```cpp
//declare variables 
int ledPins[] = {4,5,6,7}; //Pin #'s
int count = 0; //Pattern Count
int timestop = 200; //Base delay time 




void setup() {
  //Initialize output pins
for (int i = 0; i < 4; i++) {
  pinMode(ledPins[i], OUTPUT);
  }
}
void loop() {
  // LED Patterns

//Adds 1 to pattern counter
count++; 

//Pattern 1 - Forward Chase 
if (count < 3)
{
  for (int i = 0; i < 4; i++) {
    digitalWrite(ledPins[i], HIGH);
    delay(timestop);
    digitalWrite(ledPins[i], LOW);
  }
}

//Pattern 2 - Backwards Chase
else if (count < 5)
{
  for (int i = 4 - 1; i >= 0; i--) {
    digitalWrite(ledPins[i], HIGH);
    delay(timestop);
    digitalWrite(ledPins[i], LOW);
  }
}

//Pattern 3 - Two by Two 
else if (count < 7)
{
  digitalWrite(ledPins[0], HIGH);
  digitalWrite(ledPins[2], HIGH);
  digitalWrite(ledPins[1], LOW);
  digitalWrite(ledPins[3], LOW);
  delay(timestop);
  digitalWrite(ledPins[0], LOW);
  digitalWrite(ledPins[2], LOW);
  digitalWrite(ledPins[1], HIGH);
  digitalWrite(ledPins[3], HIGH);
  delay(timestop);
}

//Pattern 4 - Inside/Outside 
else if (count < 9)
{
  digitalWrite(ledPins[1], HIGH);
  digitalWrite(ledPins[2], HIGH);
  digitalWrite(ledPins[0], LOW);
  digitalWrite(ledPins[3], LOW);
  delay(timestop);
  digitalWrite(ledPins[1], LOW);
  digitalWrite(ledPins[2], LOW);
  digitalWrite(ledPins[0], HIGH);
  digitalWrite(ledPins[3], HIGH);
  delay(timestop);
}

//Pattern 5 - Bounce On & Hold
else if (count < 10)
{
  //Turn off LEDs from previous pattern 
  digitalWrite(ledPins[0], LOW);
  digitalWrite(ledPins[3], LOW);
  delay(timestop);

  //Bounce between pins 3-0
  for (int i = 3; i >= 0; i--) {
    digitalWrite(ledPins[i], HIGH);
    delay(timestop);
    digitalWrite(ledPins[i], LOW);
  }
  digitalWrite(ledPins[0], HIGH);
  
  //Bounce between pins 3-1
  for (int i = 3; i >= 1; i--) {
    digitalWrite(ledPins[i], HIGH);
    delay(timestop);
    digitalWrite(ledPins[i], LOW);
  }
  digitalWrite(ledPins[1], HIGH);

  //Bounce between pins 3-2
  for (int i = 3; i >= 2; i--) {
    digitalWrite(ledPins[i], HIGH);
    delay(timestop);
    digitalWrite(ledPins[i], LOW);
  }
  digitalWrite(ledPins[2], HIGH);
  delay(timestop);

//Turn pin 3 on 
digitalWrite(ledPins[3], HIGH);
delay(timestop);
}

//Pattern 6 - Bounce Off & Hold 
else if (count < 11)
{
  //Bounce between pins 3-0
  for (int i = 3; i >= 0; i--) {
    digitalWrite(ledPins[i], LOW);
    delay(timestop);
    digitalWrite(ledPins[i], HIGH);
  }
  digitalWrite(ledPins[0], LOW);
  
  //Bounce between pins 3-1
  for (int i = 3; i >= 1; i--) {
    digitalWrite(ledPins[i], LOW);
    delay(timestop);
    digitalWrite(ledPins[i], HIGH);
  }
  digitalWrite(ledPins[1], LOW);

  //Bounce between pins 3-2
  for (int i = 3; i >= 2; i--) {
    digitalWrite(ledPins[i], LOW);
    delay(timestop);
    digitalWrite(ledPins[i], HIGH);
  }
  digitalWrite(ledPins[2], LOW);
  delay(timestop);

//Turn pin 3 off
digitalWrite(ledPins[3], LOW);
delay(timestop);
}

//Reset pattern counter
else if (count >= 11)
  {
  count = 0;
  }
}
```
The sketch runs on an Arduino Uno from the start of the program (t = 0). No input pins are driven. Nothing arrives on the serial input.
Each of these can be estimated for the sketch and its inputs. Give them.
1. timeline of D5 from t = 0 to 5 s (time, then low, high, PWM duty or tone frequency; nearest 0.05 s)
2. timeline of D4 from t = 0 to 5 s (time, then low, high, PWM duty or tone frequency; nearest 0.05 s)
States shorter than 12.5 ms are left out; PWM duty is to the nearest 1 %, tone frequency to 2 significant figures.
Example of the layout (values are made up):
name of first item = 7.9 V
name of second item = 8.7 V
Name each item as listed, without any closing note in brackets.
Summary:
timeline of D5 from t = 0 to 5 s = 0 s low; 0.2 s high; 0.4 s low; 1 s high; 1.2 s low; 2 s high; 2.2 s low; 2.8 s high; 3 s low; 3.4 s high; 3.6 s low; 3.8 s high; 4.2 s low; 4.4 s high; 4.6 s low
timeline of D4 from t = 0 to 5 s = 0 s high; 0.2 s low; 0.8 s high; 1 s low; 2.2 s high; 2.4 s low; 3 s high; 3.4 s low; 3.6 s high; 3.8 s low; 4.2 s high; 4.4 s low; 4.6 s high; 4.8 s low
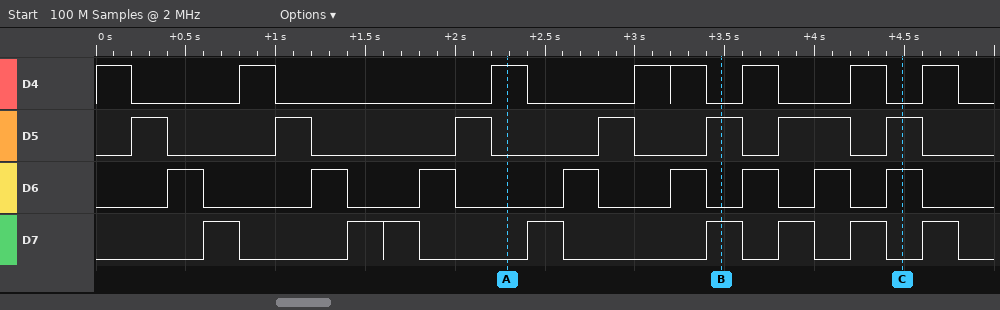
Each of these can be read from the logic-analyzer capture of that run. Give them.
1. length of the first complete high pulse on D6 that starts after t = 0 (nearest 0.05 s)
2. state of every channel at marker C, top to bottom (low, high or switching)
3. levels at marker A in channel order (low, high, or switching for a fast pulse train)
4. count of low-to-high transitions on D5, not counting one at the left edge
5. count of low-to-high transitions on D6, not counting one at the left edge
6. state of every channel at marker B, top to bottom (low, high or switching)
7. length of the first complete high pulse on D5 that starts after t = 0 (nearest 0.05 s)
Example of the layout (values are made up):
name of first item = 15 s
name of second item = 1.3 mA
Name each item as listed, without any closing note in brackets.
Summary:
length of the first complete high pulse on D6 that starts after t = 0 = 0.20 s
state of every channel at marker C, top to bottom = D4 low, D5 high, D6 high, D7 low
levels at marker A in channel order = D4 high, D5 low, D6 low, D7 low
count of low-to-high transitions on D5, not counting one at the left edge = 7
count of low-to-high transitions on D6, not counting one at the left edge = 8
state of every channel at marker B, top to bottom = D4 low, D5 high, D6 low, D7 high
length of the first complete high pulse on D5 that starts after t = 0 = 0.20 s
